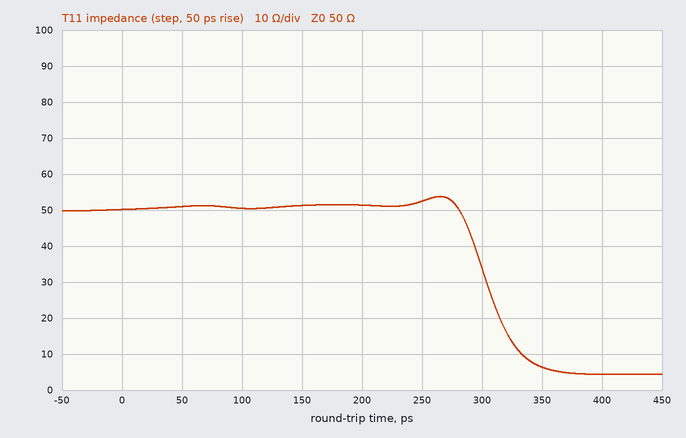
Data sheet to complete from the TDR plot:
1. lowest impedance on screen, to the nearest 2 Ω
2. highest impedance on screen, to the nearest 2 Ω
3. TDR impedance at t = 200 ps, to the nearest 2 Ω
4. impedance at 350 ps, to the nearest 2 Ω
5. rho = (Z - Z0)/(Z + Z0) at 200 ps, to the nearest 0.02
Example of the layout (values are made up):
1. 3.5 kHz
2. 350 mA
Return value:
1. 4 Ω
2. 54 Ω
3. 52 Ω
4. 6 Ω
5. +0.02
